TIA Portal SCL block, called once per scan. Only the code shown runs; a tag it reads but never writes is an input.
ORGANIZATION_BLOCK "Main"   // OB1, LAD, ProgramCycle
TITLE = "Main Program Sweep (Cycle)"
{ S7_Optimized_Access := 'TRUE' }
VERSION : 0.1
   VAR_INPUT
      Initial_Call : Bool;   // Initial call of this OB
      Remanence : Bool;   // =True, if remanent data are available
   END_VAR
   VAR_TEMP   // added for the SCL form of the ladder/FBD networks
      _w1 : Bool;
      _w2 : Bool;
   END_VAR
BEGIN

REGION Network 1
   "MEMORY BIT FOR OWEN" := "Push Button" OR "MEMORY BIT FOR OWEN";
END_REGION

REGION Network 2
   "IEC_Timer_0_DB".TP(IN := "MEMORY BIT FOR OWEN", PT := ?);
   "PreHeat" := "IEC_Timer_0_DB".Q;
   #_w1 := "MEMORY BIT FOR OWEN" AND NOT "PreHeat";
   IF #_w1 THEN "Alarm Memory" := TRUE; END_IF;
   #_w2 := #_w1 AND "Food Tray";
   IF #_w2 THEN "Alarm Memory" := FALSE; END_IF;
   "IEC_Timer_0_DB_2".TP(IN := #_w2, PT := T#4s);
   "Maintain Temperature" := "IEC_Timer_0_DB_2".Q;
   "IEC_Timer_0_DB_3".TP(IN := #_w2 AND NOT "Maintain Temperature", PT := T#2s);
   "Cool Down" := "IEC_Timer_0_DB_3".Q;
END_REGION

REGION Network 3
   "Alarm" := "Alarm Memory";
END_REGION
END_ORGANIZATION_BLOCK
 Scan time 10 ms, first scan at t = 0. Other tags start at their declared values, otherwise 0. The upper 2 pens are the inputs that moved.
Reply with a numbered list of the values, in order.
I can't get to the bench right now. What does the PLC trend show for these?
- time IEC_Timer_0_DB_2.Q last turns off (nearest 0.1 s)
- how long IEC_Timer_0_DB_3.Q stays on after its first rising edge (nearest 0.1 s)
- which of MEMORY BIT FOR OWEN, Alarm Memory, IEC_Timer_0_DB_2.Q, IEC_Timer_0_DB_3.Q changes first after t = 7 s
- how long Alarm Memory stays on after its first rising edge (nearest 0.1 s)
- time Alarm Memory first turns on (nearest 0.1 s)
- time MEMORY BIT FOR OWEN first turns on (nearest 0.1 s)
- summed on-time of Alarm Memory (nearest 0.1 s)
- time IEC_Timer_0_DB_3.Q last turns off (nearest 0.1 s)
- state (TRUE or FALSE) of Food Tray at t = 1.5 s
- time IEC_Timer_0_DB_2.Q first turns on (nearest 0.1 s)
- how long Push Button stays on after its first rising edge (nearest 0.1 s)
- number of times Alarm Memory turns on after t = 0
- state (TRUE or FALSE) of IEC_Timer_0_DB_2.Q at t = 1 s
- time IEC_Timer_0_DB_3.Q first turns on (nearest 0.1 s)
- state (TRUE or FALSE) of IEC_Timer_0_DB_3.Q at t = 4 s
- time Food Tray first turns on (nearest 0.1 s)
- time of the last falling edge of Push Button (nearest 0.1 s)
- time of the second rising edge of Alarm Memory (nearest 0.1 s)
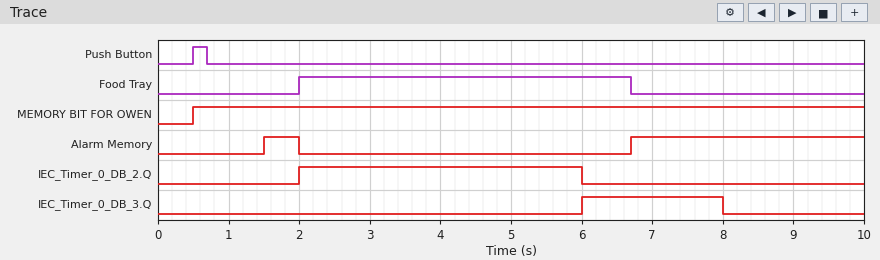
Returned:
1. 6.0 s
2. 2.0 s
3. IEC_Timer_0_DB_3.Q
4. 0.5 s
5. 1.5 s
6. 0.5 s
7. 3.8 s
8. 8.0 s
9. FALSE
10. 2.0 s
11. 0.2 s
12. 2
13. FALSE
14. 6.0 s
15. FALSE
16. 2.0 s
17. 0.7 s
18. 6.7 s
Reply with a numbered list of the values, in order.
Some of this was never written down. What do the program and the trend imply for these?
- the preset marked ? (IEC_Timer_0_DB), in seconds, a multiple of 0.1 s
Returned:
1. 1.0 s
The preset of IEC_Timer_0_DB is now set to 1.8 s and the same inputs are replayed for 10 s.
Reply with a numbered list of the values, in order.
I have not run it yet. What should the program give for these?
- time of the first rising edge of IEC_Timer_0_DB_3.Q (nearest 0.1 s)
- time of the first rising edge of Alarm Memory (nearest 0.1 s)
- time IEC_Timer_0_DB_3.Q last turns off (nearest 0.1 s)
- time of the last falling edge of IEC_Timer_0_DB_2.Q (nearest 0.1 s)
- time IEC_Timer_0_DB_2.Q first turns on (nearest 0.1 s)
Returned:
1. 6.3 s
2. 6.7 s
3. 8.3 s
4. 6.3 s
5. 2.3 s
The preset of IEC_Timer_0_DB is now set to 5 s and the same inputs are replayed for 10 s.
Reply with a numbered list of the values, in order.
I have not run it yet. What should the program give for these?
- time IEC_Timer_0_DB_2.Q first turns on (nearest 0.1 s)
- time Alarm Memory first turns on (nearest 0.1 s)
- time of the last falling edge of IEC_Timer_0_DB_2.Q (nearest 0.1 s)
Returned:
1. 5.5 s
2. 6.7 s
3. 9.5 s
